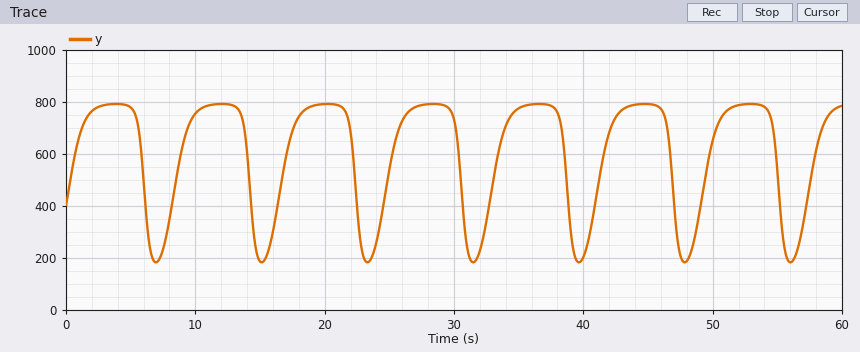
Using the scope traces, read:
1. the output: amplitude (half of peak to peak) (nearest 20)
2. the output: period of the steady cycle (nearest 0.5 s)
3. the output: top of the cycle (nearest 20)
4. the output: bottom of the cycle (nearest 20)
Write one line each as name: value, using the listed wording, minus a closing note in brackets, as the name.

the output: amplitude (half of peak to peak): 300
the output: period of the steady cycle: 8.0 s
the output: top of the cycle: 800
the output: bottom of the cycle: 180
